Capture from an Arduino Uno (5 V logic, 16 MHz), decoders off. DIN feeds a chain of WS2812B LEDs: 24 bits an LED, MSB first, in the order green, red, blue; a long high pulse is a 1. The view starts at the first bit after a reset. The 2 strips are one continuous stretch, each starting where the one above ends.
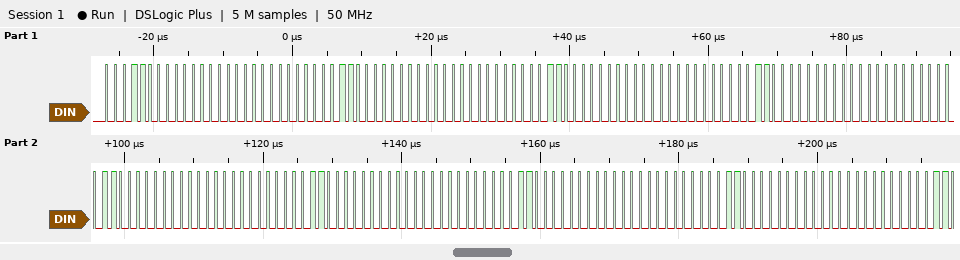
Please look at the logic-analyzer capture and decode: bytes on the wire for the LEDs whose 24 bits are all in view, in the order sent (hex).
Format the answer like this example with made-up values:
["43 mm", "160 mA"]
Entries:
["18 00 00 18 00 00 18 00 00 18 00 00 18 00 00 18 00 00 18 00 00 18 00 00"]
